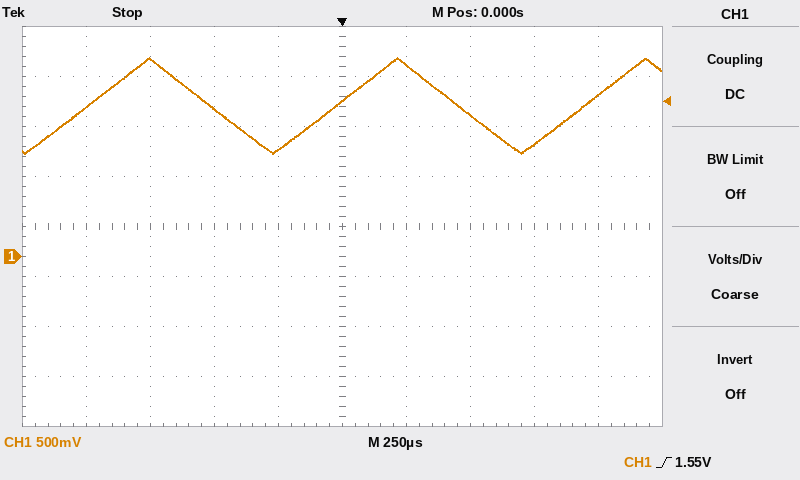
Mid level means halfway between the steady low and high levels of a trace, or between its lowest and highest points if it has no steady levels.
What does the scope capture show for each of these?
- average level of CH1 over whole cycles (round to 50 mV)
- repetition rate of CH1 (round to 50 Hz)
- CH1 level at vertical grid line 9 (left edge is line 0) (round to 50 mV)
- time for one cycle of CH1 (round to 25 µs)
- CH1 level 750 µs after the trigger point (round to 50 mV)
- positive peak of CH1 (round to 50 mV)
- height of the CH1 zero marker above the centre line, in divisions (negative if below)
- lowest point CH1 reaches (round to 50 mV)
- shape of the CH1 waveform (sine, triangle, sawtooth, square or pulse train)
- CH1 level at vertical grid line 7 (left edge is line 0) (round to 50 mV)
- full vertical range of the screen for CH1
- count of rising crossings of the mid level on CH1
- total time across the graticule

1.50 V
1.05 kHz
1.60 V
975 µs
1.10 V
2.00 V
-0.6 div
1.00 V
triangle
1.40 V
4 V
3
2.5 ms
